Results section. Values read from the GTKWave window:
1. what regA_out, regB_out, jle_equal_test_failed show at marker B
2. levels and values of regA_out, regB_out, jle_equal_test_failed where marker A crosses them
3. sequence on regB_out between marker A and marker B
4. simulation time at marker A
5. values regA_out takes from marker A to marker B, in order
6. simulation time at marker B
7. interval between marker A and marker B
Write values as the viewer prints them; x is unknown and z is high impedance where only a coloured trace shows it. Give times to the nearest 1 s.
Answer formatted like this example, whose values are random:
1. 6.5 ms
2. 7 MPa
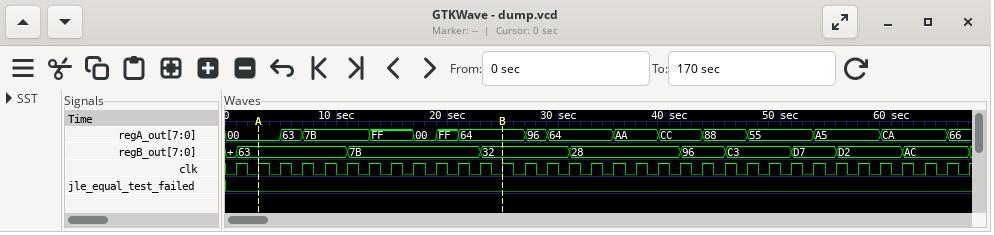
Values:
1. regA_out=64, regB_out=32, jle_equal_test_failed=0
2. regA_out=00, regB_out=63, jle_equal_test_failed=0
3. 63, 7B, 32
4. 3 s
5. 00, 63, 7B, FF, 00, FF, 64
6. 25 s
7. 22 s
